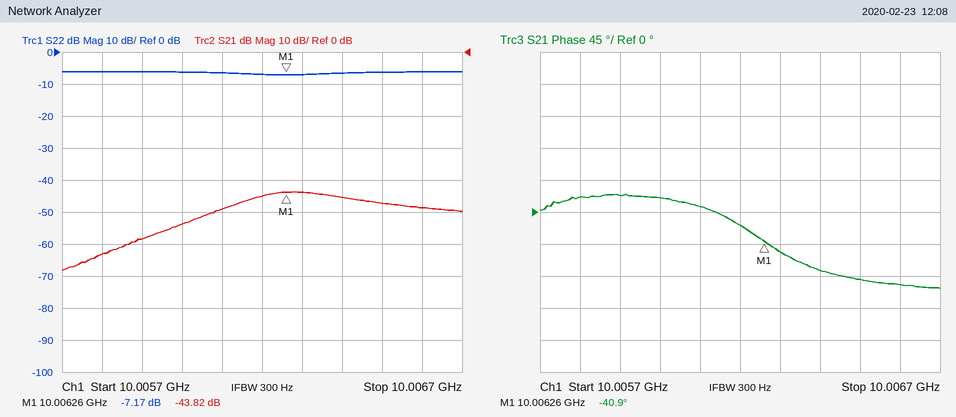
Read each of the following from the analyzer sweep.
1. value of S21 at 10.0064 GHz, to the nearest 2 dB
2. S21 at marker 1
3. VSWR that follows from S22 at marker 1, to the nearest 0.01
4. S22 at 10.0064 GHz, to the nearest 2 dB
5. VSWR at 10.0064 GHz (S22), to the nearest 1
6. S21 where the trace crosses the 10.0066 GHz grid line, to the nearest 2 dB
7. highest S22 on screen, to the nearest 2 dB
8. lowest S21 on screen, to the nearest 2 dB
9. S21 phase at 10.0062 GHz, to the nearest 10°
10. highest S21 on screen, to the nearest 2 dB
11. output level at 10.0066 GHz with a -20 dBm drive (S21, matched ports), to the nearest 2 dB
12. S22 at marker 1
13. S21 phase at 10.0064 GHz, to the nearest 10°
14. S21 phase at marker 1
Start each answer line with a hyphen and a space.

- -46 dB
- -43.82 dB
- 2.56
- -6 dB
- 3
- -48 dB
- -6 dB
- -68 dB
- -20°
- -44 dB
- -68 dBm
- -7.17 dB
- -80°
- -40.9°
